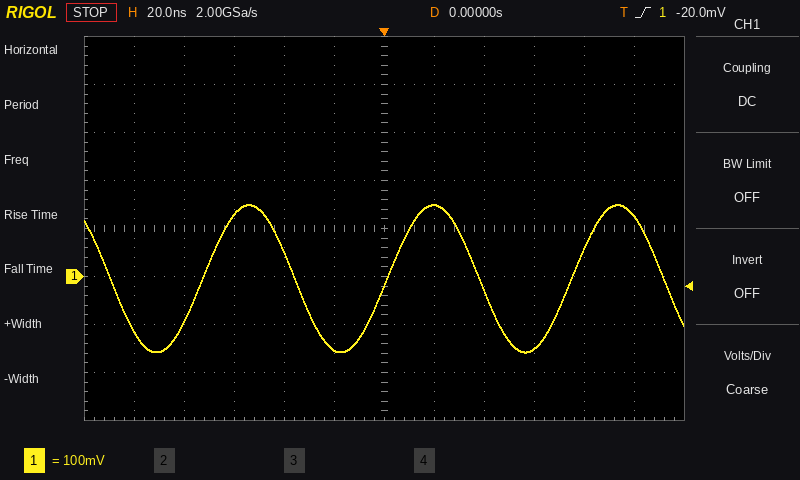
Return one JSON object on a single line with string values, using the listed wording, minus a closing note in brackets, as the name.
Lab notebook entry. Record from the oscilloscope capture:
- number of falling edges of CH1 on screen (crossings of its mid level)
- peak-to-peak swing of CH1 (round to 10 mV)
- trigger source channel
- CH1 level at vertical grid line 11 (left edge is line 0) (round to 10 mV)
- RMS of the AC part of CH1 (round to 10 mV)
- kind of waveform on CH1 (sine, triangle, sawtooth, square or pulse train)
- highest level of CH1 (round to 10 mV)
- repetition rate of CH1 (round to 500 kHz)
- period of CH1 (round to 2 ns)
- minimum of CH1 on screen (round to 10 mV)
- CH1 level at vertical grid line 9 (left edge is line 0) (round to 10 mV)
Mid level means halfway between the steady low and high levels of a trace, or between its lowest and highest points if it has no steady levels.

{"number of falling edges of CH1 on screen": "4", "peak-to-peak swing of CH1": "310 mV", "trigger source channel": "CH1", "CH1 level at vertical grid line 11 (left edge is line 0)": "130 mV", "RMS of the AC part of CH1": "110 mV", "kind of waveform on CH1": "sine", "highest level of CH1": "150 mV", "repetition rate of CH1": "13.5 MHz", "period of CH1": "74 ns", "minimum of CH1 on screen": "-160 mV", "CH1 level at vertical grid line 9 (left edge is line 0)": "-150 mV"}
